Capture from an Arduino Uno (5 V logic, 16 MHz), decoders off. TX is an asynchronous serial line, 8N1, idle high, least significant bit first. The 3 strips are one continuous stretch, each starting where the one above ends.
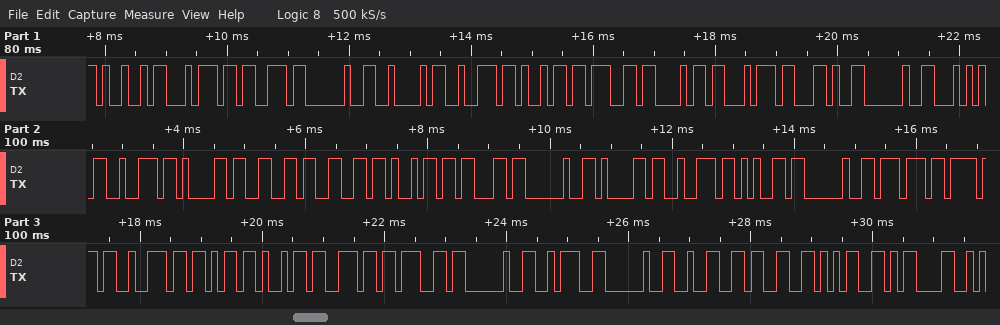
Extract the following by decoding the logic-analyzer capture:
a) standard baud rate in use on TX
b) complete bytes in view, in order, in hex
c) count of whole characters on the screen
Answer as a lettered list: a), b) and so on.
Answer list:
a) 9600 baud
b) 49 74 73 20 42 72 69 67 68 74 2C 20 54 72 61 66 66 69 63 20 61 72 65 20 77 6F 72 6B 69 6E 67 20 3A 20 32 33 35 0D
c) 38
